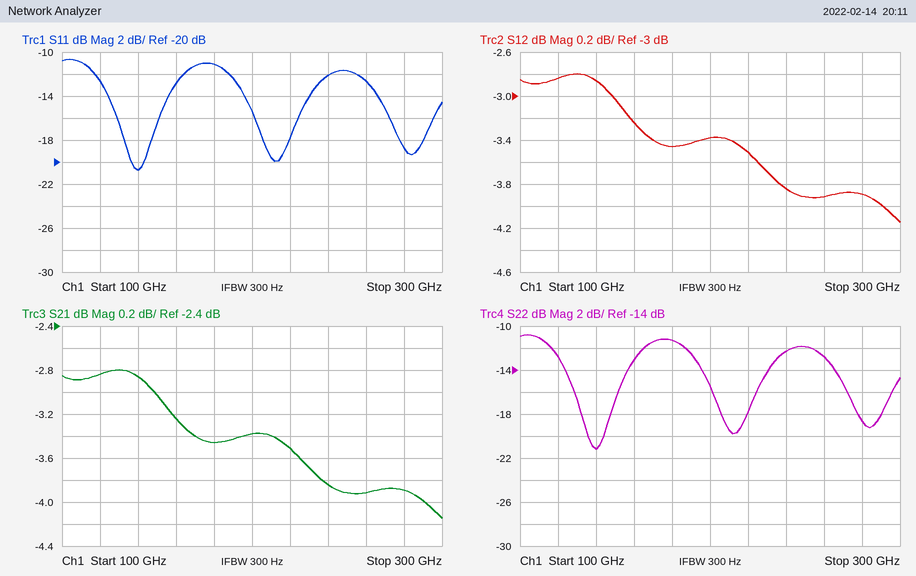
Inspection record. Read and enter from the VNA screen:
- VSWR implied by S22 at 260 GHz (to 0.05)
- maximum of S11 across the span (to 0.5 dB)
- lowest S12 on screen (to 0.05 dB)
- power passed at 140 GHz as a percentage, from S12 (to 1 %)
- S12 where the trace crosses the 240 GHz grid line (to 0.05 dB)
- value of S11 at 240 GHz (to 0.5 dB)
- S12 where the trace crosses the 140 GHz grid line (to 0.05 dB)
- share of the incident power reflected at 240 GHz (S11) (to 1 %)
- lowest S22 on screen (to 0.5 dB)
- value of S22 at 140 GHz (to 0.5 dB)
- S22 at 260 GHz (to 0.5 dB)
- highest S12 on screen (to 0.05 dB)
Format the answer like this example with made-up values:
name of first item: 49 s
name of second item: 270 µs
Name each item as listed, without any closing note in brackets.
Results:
VSWR implied by S22 at 260 GHz: 1.60
maximum of S11 across the span: -10.5 dB
lowest S12 on screen: -4.15 dB
power passed at 140 GHz as a percentage, from S12: 52 %
S12 where the trace crosses the 240 GHz grid line: -3.85 dB
value of S11 at 240 GHz: -12.0 dB
S12 where the trace crosses the 140 GHz grid line: -2.85 dB
share of the incident power reflected at 240 GHz (S11): 6 %
lowest S22 on screen: -21.0 dB
value of S22 at 140 GHz: -21.0 dB
S22 at 260 GHz: -13.0 dB
highest S12 on screen: -2.80 dB
